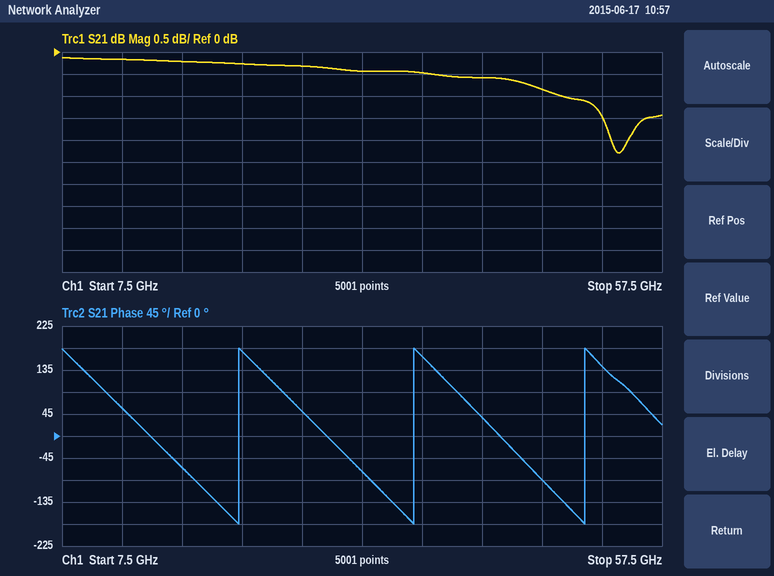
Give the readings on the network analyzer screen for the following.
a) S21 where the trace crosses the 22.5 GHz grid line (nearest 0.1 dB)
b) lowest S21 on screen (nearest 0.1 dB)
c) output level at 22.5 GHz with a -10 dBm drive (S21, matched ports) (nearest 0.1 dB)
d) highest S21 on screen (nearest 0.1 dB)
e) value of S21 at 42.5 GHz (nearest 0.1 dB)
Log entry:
-0.3 dB
-2.3 dB
-10.3 dBm
-0.1 dB
-0.6 dB
